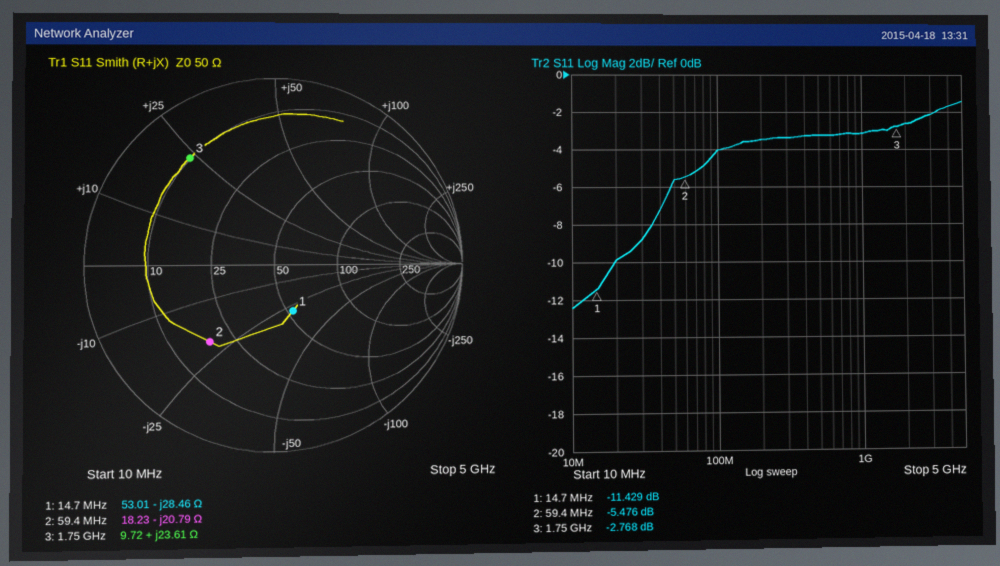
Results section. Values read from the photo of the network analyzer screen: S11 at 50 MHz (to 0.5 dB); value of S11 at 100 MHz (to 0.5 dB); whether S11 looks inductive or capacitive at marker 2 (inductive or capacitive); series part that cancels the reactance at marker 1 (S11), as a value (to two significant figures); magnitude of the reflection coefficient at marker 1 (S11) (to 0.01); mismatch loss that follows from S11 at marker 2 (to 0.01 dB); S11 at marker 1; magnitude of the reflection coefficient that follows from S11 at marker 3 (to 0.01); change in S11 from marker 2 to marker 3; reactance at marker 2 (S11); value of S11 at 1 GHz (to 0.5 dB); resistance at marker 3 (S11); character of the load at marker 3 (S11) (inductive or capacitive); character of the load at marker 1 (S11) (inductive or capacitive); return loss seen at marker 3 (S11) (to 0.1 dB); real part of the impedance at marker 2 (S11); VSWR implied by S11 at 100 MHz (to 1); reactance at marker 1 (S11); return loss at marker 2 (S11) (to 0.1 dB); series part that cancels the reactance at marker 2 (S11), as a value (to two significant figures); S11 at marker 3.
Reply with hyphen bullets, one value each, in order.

- -5.5 dB
- -4.0 dB
- capacitive
- 310 nH
- 0.27
- 1.45 dB
- -11.429 dB
- 0.73
- 2.708 dB
- -20.79 Ω
- -3.0 dB
- 9.72 Ω
- inductive
- capacitive
- 2.8 dB
- 18.23 Ω
- 4
- -28.46 Ω
- 5.5 dB
- 56 nH
- -2.768 dB
